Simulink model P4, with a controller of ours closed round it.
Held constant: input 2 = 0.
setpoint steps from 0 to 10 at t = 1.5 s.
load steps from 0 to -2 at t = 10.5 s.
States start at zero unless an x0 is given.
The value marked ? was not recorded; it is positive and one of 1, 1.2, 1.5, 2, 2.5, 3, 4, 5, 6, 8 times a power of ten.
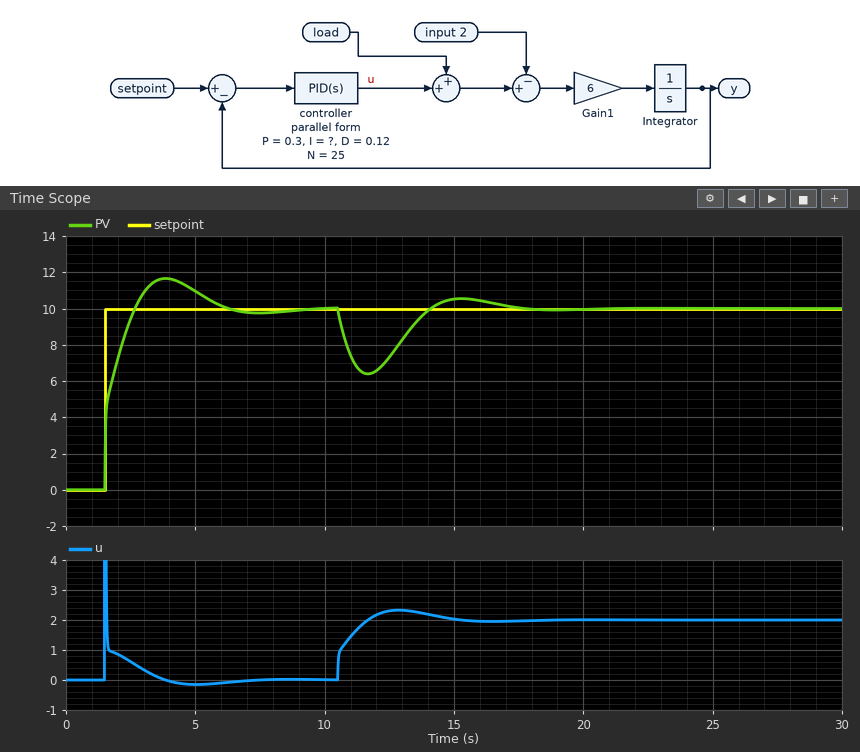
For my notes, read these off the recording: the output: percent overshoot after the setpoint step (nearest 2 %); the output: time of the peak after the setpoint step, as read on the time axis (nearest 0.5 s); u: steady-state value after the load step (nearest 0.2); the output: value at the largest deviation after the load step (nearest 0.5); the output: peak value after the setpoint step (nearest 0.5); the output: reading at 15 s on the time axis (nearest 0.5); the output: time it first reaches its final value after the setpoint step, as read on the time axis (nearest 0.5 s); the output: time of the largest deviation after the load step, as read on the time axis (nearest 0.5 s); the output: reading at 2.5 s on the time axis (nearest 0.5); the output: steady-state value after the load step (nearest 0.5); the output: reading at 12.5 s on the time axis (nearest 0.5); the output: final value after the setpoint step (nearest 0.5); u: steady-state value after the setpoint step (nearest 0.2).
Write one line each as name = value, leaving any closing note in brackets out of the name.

the output: percent overshoot after the setpoint step = 16 %
the output: time of the peak after the setpoint step, as read on the time axis = 4.0 s
u: steady-state value after the load step = 2.0
the output: value at the largest deviation after the load step = 6.5
the output: peak value after the setpoint step = 11.5
the output: reading at 15 s on the time axis = 10.5
the output: time it first reaches its final value after the setpoint step, as read on the time axis = 2.5 s
the output: time of the largest deviation after the load step, as read on the time axis = 11.5 s
the output: reading at 2.5 s on the time axis = 9.5
the output: steady-state value after the load step = 10.0
the output: reading at 12.5 s on the time axis = 7.5
the output: final value after the setpoint step = 10.0
u: steady-state value after the setpoint step = 0.0
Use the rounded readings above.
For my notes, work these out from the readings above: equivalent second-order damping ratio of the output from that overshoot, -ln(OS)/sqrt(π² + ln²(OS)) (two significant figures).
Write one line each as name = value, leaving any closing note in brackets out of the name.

equivalent second-order damping ratio of the output from that overshoot, -ln(OS)/sqrt(π² + ln²(OS)) = 0.50
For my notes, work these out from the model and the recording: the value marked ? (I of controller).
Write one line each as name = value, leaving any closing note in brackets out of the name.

the value marked ? = 0.3
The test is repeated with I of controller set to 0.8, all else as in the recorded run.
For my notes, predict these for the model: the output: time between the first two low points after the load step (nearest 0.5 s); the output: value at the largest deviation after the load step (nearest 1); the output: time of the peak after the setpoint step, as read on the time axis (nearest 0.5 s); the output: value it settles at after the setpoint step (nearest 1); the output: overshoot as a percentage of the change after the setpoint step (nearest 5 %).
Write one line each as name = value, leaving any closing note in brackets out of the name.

the output: time between the first two low points after the load step = 4.0 s
the output: value at the largest deviation after the load step = 7
the output: time of the peak after the setpoint step, as read on the time axis = 3.0 s
the output: value it settles at after the setpoint step = 10
the output: overshoot as a percentage of the change after the setpoint step = 25 %
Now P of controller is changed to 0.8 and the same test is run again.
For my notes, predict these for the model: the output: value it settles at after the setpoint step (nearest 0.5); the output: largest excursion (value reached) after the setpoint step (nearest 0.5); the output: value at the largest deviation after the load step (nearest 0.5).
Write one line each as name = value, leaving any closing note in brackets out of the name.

the output: value it settles at after the setpoint step = 10.0
the output: largest excursion (value reached) after the setpoint step = 10.5
the output: value at the largest deviation after the load step = 8.0
